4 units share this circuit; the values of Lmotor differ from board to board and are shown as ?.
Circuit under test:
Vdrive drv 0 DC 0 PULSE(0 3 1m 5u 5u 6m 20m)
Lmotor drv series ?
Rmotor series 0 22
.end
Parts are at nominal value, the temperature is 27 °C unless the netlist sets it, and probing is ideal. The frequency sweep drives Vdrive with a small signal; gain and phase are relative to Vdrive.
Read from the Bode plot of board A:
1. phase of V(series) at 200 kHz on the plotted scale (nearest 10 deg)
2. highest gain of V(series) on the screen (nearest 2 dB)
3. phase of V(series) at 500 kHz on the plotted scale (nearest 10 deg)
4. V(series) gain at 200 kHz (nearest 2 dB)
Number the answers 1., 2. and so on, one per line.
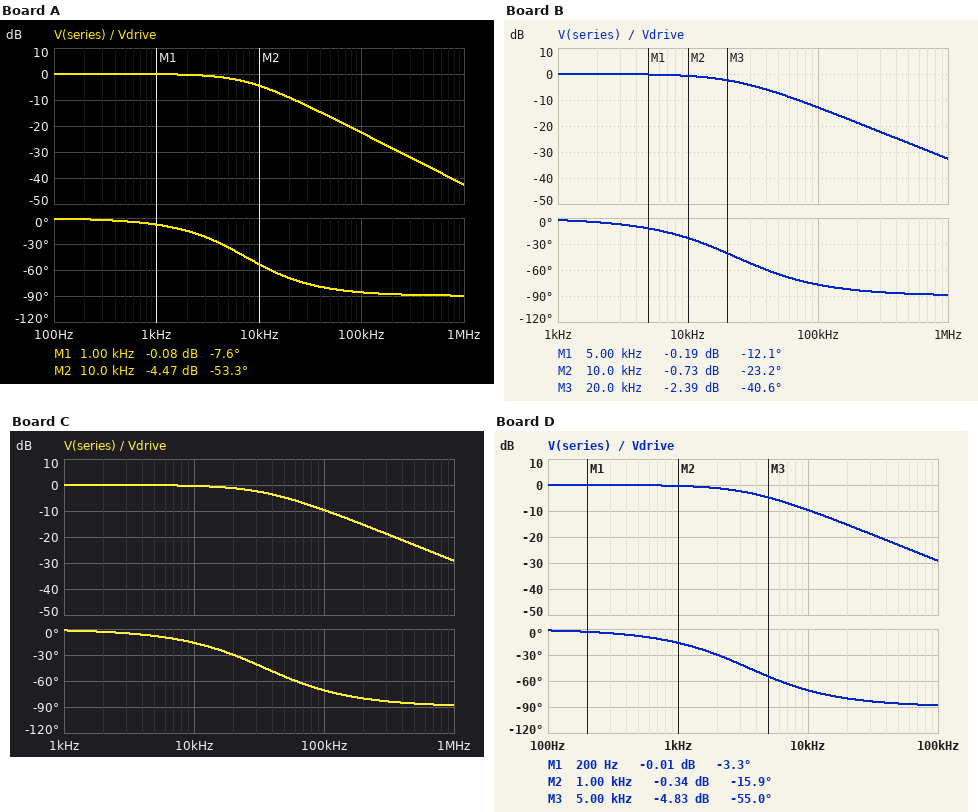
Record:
1. -90 deg
2. 0 dB
3. -90 deg
4. -28 dB
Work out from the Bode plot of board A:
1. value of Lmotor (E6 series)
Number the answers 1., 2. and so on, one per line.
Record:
1. 470 µH
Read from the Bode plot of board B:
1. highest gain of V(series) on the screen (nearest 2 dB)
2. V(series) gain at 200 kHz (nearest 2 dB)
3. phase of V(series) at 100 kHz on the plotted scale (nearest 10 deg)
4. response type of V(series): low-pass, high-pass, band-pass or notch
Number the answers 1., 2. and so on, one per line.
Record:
1. 0 dB
2. -18 dB
3. -80 deg
4. low-pass
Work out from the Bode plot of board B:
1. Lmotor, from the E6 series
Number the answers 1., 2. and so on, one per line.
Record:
1. 150 µH
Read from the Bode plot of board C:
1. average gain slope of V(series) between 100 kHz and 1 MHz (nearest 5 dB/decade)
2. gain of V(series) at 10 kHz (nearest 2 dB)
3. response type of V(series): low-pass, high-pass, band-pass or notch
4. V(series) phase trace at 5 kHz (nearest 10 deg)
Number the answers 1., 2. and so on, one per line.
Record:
1. -20 dB/decade
2. 0 dB
3. low-pass
4. -10 deg
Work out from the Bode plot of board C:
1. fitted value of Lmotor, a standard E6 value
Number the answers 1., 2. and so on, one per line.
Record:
1. 100 µH
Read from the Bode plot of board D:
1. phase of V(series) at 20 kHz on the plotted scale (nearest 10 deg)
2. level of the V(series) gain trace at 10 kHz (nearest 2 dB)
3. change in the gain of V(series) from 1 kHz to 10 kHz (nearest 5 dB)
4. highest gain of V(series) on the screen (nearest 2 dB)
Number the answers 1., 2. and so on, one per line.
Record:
1. -80 deg
2. -10 dB
3. -10 dB
4. 0 dB
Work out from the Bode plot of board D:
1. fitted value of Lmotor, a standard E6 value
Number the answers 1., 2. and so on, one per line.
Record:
1. 1 mH
